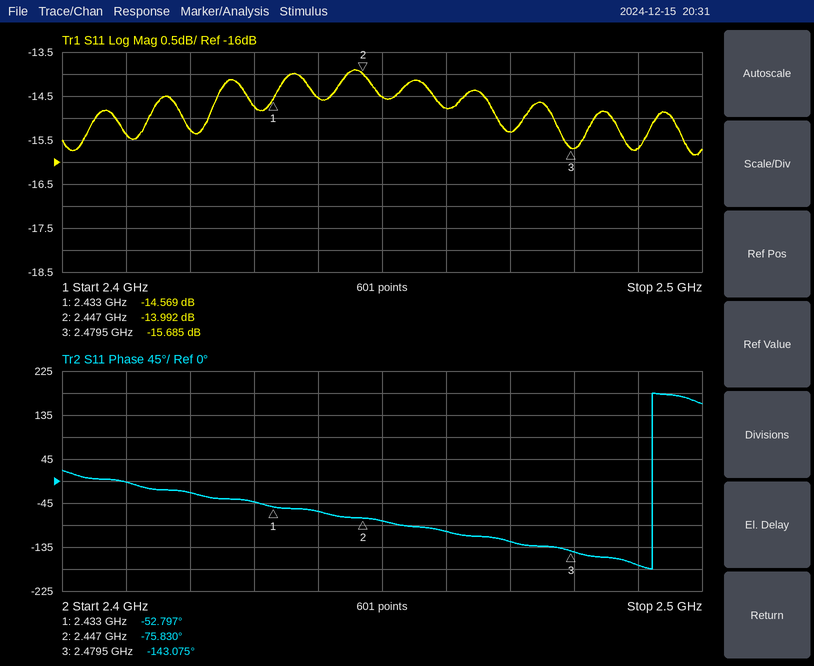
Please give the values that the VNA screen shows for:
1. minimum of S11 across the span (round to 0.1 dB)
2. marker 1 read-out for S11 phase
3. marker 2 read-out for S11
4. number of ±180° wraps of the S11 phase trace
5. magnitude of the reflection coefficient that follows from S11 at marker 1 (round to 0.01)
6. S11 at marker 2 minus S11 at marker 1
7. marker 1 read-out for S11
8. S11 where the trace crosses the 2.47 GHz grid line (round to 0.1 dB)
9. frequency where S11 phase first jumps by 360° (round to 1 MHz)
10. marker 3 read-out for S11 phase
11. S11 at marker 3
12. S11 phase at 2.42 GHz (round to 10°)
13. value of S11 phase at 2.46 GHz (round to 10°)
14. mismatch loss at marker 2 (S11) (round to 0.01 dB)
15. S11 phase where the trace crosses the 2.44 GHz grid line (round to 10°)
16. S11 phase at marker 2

-15.8 dB
-52.797°
-13.992 dB
1
0.19
0.577 dB
-14.569 dB
-15.3 dB
2.492 GHz
-143.075°
-15.685 dB
-20°
-100°
0.18 dB
-60°
-75.830°
